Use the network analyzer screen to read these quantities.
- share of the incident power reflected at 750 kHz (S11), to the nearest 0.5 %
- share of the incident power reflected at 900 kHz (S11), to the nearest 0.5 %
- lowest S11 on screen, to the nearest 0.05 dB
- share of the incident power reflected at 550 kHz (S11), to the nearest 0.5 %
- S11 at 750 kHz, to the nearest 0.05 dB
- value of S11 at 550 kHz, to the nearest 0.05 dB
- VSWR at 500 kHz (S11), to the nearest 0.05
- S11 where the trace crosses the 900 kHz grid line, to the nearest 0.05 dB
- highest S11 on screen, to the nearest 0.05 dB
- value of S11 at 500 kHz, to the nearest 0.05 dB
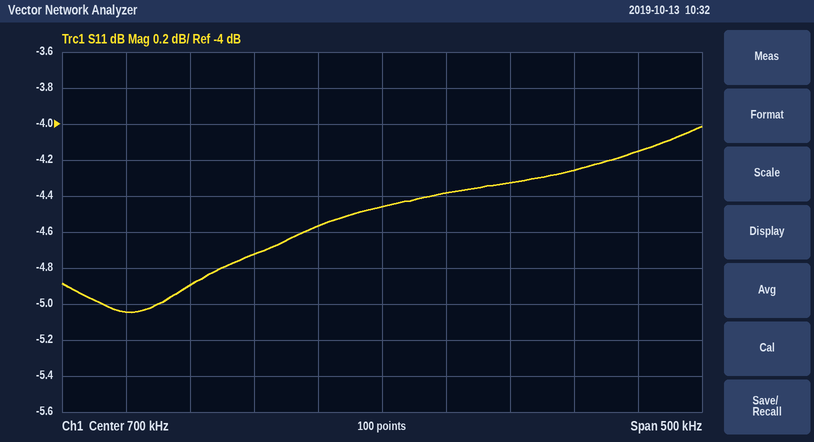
36.5 %
38.5 %
-5.05 dB
32.5 %
-4.40 dB
-4.90 dB
3.55
-4.15 dB
-4.00 dB
-5.05 dB
